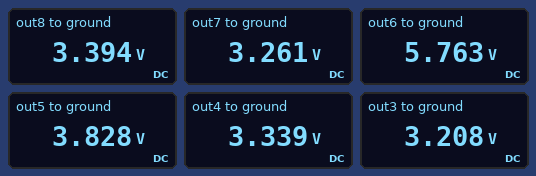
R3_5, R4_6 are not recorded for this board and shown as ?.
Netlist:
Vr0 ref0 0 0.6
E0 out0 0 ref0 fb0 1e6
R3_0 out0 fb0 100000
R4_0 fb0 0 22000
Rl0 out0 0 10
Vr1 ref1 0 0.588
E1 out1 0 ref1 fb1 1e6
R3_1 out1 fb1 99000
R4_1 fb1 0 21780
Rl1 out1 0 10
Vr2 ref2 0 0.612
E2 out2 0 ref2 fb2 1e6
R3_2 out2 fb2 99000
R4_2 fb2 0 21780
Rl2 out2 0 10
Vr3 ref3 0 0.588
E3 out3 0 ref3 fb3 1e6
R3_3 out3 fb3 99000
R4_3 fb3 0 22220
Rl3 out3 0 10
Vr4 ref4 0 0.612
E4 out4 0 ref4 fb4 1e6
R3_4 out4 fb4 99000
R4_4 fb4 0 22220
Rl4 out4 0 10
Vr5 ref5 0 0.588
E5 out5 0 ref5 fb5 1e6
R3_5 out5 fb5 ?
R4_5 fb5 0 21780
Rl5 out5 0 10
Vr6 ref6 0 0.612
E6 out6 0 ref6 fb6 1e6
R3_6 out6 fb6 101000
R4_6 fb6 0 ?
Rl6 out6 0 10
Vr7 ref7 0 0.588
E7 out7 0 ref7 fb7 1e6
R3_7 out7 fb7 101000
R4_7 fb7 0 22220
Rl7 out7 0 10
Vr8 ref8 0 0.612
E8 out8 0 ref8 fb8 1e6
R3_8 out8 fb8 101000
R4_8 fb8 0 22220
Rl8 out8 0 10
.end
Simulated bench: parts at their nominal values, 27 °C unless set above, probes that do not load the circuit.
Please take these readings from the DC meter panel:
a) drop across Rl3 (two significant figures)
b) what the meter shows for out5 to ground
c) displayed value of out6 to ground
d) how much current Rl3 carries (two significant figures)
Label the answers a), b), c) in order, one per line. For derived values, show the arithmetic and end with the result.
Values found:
a) 3.208 V = 3.2 V
b) 3.828 V
c) 5.763 V
d) (3.208 V) / 10 Ω = 320 mA
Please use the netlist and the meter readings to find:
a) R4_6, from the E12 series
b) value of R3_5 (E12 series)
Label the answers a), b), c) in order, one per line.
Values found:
a) 12 kΩ
b) 120 kΩ
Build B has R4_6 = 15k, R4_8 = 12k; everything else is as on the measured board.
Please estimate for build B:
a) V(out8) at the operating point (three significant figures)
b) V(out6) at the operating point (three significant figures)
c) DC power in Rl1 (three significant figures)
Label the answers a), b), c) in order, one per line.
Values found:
a) 5.76 V
b) 4.73 V
c) 1.06 W
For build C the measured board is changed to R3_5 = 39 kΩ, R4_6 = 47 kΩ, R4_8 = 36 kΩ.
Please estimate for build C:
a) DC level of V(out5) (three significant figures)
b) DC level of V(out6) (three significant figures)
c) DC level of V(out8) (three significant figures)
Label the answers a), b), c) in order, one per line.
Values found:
a) 1.64 V
b) 1.93 V
c) 2.33 V
